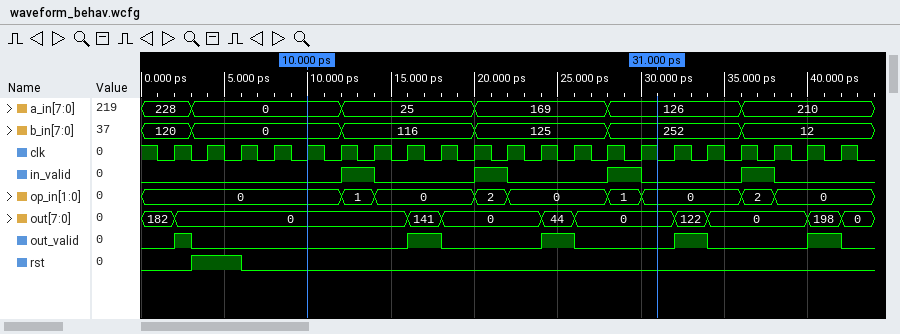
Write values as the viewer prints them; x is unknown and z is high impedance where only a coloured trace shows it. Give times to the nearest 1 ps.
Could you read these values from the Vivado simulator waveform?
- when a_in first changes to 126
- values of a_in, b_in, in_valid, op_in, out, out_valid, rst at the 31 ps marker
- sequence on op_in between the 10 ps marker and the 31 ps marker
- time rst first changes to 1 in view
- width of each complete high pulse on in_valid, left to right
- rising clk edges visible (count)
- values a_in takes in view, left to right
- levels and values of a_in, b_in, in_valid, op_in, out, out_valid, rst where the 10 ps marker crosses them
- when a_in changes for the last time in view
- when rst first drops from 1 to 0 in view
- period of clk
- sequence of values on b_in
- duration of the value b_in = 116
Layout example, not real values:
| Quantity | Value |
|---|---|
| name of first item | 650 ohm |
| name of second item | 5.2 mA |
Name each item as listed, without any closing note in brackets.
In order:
| Quantity | Value |
|---|---|
| when a_in first changes to 126 | 28 ps |
| values of a_in, b_in, in_valid, op_in, out, out_valid, rst at the 31 ps marker | a_in=126, b_in=252, in_valid=0, op_in=0, out=0, out_valid=0, rst=0 |
| sequence on op_in between the 10 ps marker and the 31 ps marker | 0, 1, 0, 2, 0, 1, 0 |
| time rst first changes to 1 in view | 3 ps |
| width of each complete high pulse on in_valid, left to right | 2 ps, 2 ps, 2 ps, 2 ps |
| rising clk edges visible | 21 |
| values a_in takes in view, left to right | 228, 0, 25, 169, 126, 210 |
| levels and values of a_in, b_in, in_valid, op_in, out, out_valid, rst where the 10 ps marker crosses them | a_in=0, b_in=0, in_valid=0, op_in=0, out=0, out_valid=0, rst=0 |
| when a_in changes for the last time in view | 36 ps |
| when rst first drops from 1 to 0 in view | 6 ps |
| period of clk | 2 ps |
| sequence of values on b_in | 120, 0, 116, 125, 252, 12 |
| duration of the value b_in = 116 | 8 ps |
